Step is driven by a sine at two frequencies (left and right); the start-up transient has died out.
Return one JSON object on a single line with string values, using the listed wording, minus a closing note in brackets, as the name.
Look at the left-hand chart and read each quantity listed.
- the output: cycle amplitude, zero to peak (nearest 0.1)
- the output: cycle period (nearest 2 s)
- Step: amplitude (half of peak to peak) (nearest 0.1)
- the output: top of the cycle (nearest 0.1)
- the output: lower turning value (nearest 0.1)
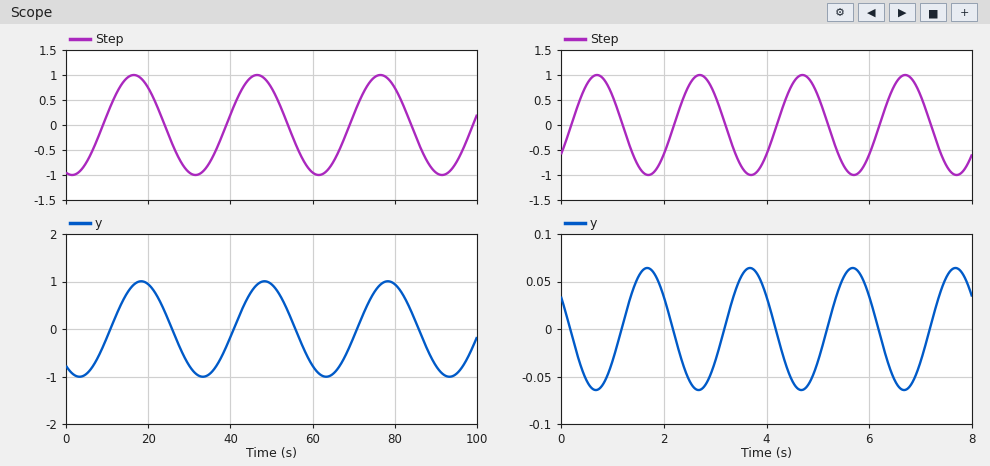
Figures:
{"the output: cycle amplitude, zero to peak": "1.0", "the output: cycle period": "30 s", "Step: amplitude (half of peak to peak)": "1.0", "the output: top of the cycle": "1.0", "the output: lower turning value": "-1.0"}
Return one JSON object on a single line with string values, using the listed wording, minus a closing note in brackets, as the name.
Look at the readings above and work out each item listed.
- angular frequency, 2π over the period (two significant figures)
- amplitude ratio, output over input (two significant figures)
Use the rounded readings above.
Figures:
{"angular frequency, 2π over the period": "0.21 rad/s", "amplitude ratio, output over input": "1.0"}
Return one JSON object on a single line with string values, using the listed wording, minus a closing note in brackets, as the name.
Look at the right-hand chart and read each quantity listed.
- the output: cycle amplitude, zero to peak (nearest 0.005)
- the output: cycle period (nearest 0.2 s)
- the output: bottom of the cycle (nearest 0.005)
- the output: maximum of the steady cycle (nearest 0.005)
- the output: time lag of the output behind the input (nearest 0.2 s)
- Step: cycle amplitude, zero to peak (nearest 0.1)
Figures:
{"the output: cycle amplitude, zero to peak": "0.065", "the output: cycle period": "2.0 s", "the output: bottom of the cycle": "-0.065", "the output: maximum of the steady cycle": "0.065", "the output: time lag of the output behind the input": "1.0 s", "Step: cycle amplitude, zero to peak": "1.0"}
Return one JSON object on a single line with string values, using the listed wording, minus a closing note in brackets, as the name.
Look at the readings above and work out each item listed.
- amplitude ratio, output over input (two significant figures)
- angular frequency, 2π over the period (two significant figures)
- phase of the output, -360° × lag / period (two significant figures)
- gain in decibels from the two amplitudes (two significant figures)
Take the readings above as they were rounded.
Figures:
{"amplitude ratio, output over input": "0.065", "angular frequency, 2π over the period": "3.1 rad/s", "phase of the output, -360° × lag / period": "-180°", "gain in decibels from the two amplitudes": "-24 dB"}
